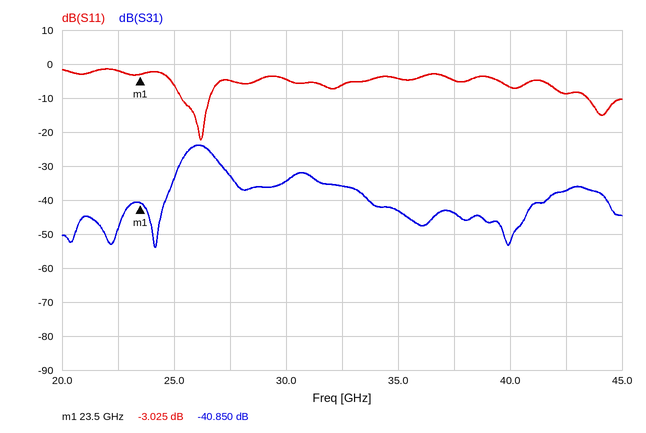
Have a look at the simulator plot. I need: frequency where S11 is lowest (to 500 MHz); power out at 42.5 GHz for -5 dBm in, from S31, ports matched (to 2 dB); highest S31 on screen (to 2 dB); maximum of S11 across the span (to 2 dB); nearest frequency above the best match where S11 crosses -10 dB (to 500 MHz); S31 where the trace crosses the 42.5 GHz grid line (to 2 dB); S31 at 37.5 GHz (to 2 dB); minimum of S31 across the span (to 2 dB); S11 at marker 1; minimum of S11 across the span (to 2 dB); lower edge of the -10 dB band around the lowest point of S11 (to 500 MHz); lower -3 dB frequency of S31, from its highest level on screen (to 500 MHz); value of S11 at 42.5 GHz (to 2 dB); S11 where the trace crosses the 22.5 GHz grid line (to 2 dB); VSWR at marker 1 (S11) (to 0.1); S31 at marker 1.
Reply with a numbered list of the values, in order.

1. 26.0 GHz
2. -42 dBm
3. -24 dB
4. -2 dB
5. 26.5 GHz
6. -38 dB
7. -44 dB
8. -54 dB
9. -3.025 dB
10. -22 dB
11. 25.5 GHz
12. 25.5 GHz
13. -8 dB
14. -2 dB
15. 5.8
16. -40.850 dB
